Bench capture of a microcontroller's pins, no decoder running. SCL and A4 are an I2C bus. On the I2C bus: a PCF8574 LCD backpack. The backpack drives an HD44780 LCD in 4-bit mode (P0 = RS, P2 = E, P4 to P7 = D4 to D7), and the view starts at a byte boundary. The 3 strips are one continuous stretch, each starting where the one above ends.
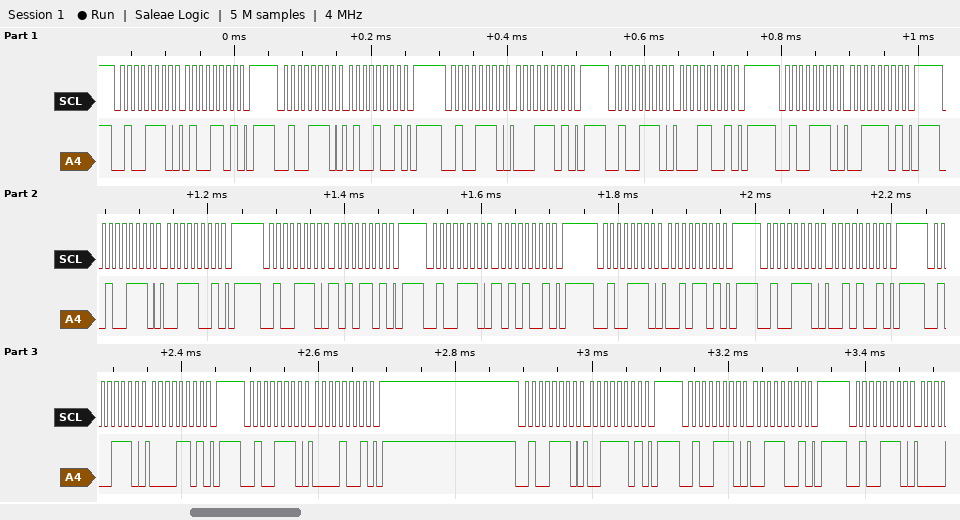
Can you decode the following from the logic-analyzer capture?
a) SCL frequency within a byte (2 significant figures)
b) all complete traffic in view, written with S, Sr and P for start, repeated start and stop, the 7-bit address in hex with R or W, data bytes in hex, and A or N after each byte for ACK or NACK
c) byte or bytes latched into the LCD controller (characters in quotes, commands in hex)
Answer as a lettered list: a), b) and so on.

a) 100 kHz
b) S 27W A 4D A P S 27W A 49 A P S 27W A 1D A P S 27W A 19 A P S 27W A 3D A P S 27W A 39 A P S 27W A AD A P S 27W A A9 A P S 27W A 2D A P S 27W A 29 A P S 27W A 0D A P S 27W A 09 A P S 27W A 3D A P S 27W A 39 A P S 27W A
c) 'A' ':' ' '
